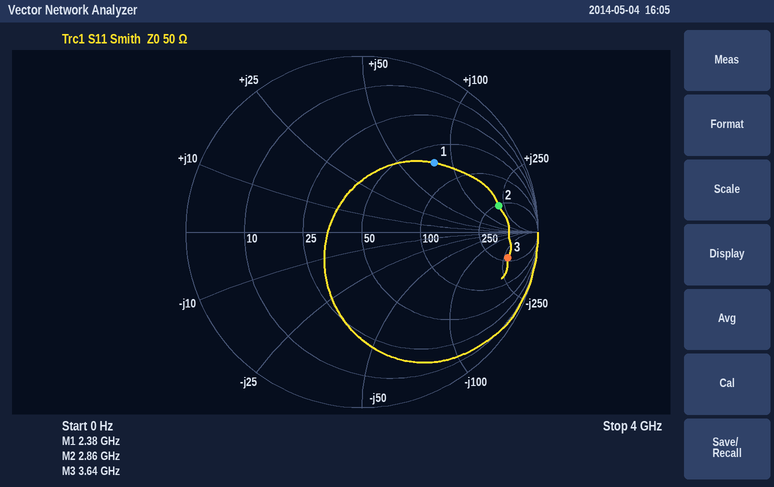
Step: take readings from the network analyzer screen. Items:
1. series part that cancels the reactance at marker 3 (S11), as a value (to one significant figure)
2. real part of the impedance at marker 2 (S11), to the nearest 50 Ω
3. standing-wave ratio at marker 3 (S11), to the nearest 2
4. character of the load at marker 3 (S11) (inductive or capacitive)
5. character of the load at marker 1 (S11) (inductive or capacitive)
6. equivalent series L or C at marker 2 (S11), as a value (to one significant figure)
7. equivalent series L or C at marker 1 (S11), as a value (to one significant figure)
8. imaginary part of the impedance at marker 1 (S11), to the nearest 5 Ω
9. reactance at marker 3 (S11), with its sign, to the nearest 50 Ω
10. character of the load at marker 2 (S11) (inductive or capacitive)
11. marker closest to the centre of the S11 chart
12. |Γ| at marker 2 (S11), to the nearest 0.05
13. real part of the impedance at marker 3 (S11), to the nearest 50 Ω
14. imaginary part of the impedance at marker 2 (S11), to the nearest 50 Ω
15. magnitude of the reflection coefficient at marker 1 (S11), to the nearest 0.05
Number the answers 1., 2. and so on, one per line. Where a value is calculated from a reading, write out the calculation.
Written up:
1. L = 300 Ω/(2π × 3.64 GHz) ≈ 13.1 nH, so 10 nH to one significant figure
2. 250 Ω
3. 12
4. capacitive
5. inductive
6. L = 200 Ω/(2π × 2.86 GHz) ≈ 11.1 nH, so 10 nH to one significant figure
7. L = 80 Ω/(2π × 2.38 GHz) ≈ 5 nH
8. +80 Ω
9. -300 Ω
10. inductive
11. marker 1
12. 0.80
13. 300 Ω
14. +200 Ω
15. 0.55
